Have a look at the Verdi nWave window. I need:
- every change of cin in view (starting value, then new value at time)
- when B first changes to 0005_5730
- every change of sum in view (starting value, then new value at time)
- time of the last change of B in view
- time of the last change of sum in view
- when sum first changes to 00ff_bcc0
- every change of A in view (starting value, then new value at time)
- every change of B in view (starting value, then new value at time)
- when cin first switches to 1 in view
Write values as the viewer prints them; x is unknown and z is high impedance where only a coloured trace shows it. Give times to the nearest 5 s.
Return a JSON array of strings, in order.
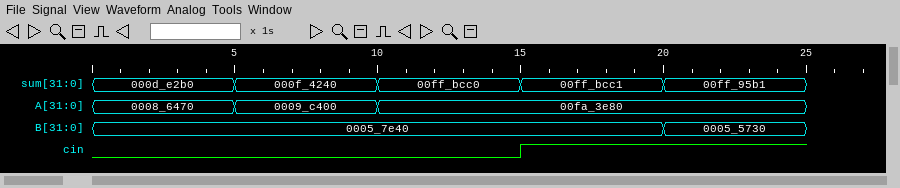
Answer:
["0, 1 at 15 s", "20 s", "000d_e2b0, 000f_4240 at 5 s, 00ff_bcc0 at 10 s, 00ff_bcc1 at 15 s, 00ff_95b1 at 20 s", "20 s", "20 s", "10 s", "0008_6470, 0009_c400 at 5 s, 00fa_3e80 at 10 s", "0005_7e40, 0005_5730 at 20 s", "15 s"]
